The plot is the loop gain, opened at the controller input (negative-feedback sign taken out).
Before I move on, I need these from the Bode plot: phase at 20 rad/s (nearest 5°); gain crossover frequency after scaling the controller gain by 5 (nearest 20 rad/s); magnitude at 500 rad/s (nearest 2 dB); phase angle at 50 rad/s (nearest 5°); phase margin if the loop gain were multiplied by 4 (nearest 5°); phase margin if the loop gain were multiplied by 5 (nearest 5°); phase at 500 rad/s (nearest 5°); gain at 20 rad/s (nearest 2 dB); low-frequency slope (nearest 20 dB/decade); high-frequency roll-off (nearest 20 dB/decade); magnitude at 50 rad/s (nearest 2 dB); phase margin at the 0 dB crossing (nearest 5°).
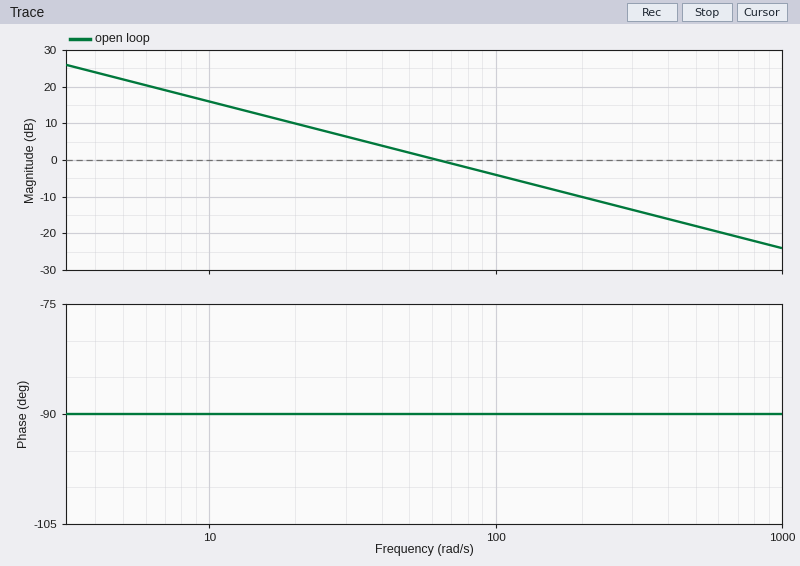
-90°
320 rad/s
-18 dB
-90°
90°
90°
-90°
10 dB
-20 dB/decade
-20 dB/decade
2 dB
90°
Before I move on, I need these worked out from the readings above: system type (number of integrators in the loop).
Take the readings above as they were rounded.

1
